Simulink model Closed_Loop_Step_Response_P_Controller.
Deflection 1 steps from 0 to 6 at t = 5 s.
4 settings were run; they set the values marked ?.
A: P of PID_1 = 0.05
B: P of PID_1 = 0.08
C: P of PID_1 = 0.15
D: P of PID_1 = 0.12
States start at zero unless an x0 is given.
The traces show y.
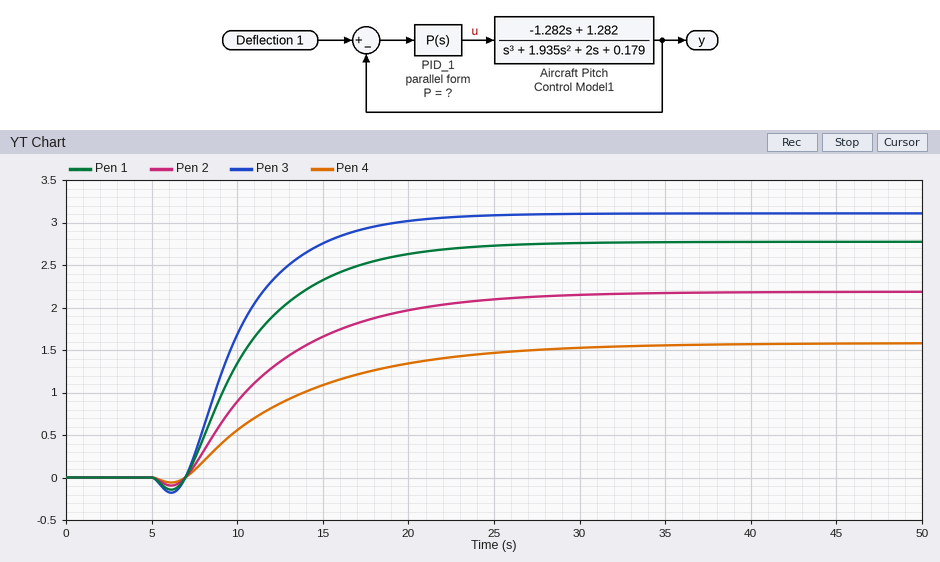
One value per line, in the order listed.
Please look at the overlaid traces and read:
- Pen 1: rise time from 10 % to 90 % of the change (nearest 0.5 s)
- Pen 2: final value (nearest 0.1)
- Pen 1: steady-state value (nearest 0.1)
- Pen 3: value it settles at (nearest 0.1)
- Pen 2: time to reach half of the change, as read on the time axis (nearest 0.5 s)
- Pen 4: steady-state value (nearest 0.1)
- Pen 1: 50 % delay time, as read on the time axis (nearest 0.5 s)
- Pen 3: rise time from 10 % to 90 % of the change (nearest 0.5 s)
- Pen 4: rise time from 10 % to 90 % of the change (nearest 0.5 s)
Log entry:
9.5 s
2.2
2.8
3.1
11.0 s
1.6
10.0 s
8.0 s
15.0 s
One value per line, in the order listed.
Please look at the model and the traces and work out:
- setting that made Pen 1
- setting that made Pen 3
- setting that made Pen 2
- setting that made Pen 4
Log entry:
D
C
B
A
